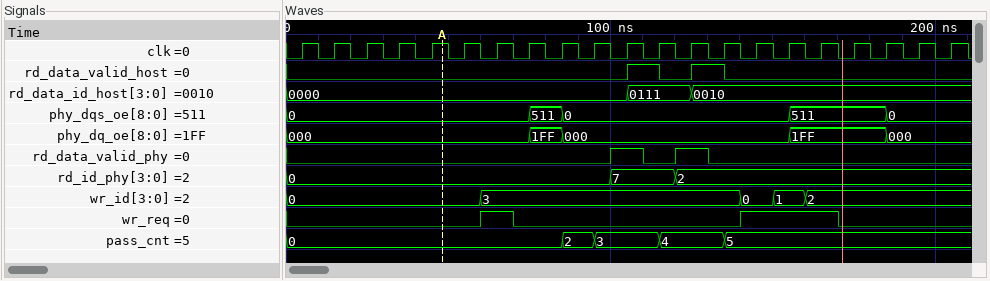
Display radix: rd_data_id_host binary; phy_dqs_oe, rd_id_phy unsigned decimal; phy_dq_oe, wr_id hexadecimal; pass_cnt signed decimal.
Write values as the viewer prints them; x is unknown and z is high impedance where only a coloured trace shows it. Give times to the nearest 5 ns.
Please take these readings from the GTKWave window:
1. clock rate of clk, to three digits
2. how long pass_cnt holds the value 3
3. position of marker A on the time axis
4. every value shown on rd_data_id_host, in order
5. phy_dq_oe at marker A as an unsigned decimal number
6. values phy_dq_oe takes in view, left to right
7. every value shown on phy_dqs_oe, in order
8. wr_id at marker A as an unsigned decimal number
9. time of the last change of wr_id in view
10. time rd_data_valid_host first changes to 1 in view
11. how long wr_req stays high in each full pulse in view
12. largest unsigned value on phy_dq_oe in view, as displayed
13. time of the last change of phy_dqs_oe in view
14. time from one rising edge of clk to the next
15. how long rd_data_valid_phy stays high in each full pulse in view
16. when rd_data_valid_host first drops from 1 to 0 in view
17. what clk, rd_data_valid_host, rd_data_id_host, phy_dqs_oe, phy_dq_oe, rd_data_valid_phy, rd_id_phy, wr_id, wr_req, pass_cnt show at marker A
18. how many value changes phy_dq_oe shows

100 MHz
20 ns
50 ns
0000, 0111, 0010
0
000, 1FF, 000, 1FF, 000
0, 511, 0, 511, 0
0
160 ns
105 ns
10 ns, 30 ns
1FF
185 ns
10 ns
10 ns, 10 ns
115 ns
clk=1, rd_data_valid_host=0, rd_data_id_host=0000, phy_dqs_oe=0, phy_dq_oe=000, rd_data_valid_phy=0, rd_id_phy=0, wr_id=0, wr_req=0, pass_cnt=0
4
